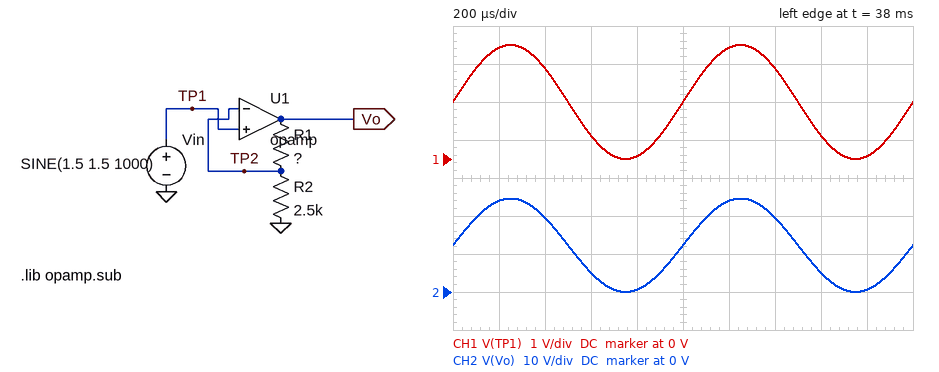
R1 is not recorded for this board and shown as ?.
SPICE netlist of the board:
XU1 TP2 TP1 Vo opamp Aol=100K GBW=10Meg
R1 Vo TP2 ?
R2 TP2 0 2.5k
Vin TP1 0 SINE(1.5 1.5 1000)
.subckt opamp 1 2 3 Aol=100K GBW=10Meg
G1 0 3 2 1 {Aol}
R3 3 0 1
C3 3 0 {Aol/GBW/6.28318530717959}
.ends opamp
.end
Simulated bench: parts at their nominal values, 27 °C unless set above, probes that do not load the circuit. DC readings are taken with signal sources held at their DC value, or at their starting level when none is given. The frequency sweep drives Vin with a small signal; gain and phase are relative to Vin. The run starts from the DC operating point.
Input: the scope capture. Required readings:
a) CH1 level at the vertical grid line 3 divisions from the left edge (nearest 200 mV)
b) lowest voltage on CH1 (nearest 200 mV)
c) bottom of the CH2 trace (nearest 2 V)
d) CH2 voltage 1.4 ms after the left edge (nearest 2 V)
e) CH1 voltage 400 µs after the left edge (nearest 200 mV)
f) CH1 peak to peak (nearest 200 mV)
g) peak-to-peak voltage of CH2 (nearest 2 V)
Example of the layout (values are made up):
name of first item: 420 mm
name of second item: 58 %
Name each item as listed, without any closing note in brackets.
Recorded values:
CH1 level at the vertical grid line 3 divisions from the left edge: 600 mV
lowest voltage on CH1: 0 V
bottom of the CH2 trace: 0 V
CH2 voltage 1.4 ms after the left edge: 20 V
CH1 voltage 400 µs after the left edge: 2.4 V
CH1 peak to peak: 3.0 V
peak-to-peak voltage of CH2: 24 V
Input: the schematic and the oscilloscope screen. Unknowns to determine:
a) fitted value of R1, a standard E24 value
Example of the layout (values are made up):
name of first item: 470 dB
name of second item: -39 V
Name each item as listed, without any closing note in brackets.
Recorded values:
fitted value of R1, a standard E24 value: 18 kΩ
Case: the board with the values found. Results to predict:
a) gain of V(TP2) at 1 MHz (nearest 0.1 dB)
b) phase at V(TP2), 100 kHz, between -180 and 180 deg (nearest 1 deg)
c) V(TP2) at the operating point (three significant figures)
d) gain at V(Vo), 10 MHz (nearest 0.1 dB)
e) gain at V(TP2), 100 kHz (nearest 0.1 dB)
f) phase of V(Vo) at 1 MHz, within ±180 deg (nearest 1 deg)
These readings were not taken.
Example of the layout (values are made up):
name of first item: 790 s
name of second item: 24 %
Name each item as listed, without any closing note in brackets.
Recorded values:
gain of V(TP2) at 1 MHz: -2.2 dB
phase at V(TP2), 100 kHz, between -180 and 180 deg: -5 deg
V(TP2) at the operating point: 1.50 V
gain at V(Vo), 10 MHz: -0.1 dB
gain at V(TP2), 100 kHz: 0 dB
phase of V(Vo) at 1 MHz, within ±180 deg: -39 deg
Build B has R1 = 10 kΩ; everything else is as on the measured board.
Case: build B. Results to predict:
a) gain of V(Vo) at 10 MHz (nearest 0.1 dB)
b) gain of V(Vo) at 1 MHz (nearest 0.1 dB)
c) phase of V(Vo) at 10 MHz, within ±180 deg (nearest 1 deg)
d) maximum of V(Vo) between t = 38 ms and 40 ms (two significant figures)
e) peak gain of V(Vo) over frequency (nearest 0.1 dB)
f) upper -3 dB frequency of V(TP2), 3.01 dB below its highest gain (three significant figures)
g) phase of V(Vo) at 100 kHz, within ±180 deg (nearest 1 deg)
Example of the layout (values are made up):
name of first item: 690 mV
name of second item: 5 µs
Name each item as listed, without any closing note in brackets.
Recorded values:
gain of V(Vo) at 10 MHz: -0.2 dB
gain of V(Vo) at 1 MHz: 13.0 dB
phase of V(Vo) at 10 MHz, within ±180 deg: -79 deg
maximum of V(Vo) between t = 38 ms and 40 ms: 15 V
peak gain of V(Vo) over frequency: 14.0 dB
upper -3 dB frequency of V(TP2), 3.01 dB below its highest gain: 2.00 MHz
phase of V(Vo) at 100 kHz, within ±180 deg: -3 deg
